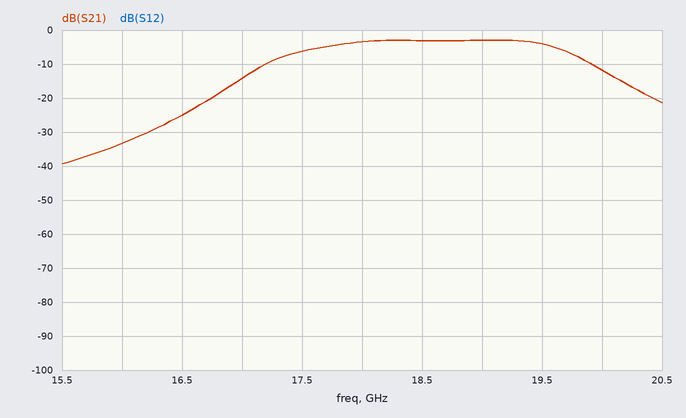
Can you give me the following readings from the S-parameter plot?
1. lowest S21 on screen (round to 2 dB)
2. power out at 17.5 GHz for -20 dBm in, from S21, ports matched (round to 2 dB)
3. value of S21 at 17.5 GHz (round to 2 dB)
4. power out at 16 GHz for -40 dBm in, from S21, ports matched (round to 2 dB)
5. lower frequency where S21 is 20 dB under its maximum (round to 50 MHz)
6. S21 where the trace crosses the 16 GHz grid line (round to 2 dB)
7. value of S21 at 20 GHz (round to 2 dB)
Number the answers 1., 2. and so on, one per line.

1. -40 dB
2. -26 dBm
3. -6 dB
4. -74 dBm
5. 16.60 GHz
6. -34 dB
7. -12 dB
